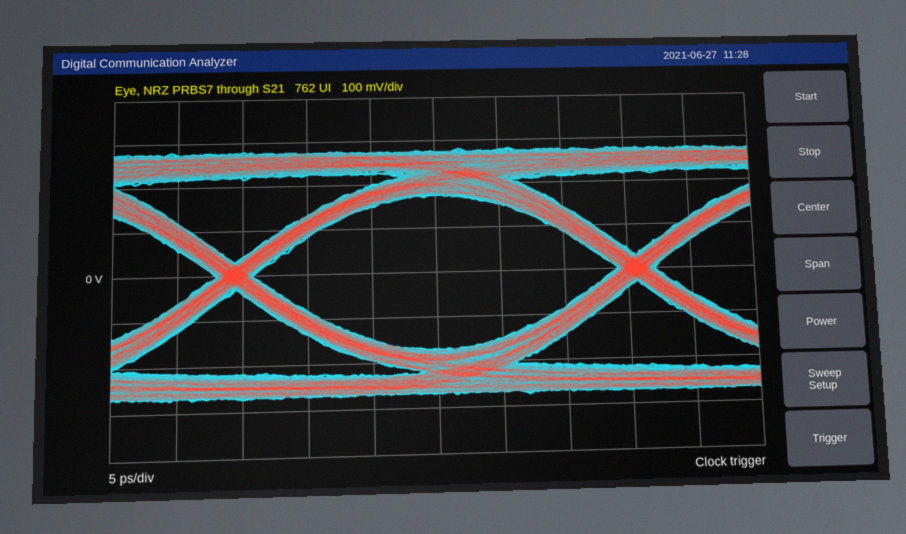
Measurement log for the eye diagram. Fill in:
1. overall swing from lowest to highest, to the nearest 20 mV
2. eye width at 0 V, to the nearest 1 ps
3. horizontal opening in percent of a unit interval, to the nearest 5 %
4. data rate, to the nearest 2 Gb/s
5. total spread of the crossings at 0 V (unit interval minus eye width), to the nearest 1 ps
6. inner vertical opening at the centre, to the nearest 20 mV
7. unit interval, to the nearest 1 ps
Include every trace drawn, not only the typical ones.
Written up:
560 mV
28 ps
90 %
32 Gb/s
3 ps
340 mV
31 ps
